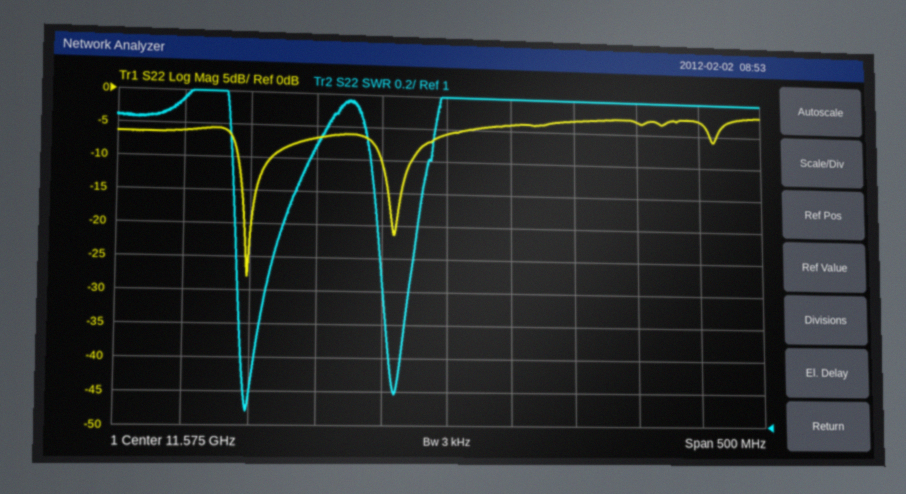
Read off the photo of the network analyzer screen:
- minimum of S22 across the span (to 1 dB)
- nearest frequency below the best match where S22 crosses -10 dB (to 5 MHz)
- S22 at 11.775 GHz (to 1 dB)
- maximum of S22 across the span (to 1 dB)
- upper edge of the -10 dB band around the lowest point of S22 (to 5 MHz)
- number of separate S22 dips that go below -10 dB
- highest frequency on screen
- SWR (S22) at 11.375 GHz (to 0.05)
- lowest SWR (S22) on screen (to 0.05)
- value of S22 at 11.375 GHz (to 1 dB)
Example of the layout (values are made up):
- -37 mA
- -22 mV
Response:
- -28 dB
- 11.415 GHz
- -3 dB
- -2 dB
- 11.440 GHz
- 2
- 11.825 GHz
- 2.95
- 1.10
- -6 dB
